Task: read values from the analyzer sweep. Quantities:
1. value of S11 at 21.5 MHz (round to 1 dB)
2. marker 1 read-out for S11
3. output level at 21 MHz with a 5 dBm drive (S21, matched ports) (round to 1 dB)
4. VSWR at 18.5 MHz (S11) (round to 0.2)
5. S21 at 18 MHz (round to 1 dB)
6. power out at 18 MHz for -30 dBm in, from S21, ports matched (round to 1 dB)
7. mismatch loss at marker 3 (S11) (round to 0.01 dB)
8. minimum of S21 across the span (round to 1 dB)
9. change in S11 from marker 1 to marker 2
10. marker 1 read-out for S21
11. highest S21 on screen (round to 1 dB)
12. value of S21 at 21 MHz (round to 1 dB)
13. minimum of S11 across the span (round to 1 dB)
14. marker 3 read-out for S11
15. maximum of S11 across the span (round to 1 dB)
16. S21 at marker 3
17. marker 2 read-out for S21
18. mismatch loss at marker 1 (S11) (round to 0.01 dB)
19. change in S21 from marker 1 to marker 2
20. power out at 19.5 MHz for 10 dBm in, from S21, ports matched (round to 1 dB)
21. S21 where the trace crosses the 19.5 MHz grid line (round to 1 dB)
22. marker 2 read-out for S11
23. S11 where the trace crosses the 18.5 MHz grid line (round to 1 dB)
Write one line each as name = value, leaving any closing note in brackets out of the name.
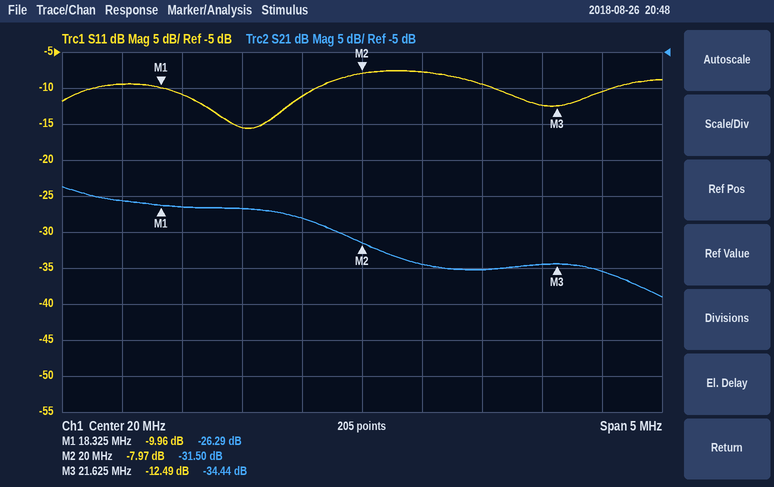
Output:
value of S11 at 21.5 MHz = -12 dB
marker 1 read-out for S11 = -9.96 dB
output level at 21 MHz with a 5 dBm drive (S21, matched ports) = -30 dBm
VSWR at 18.5 MHz (S11) = 1.8
S21 at 18 MHz = -26 dB
power out at 18 MHz for -30 dBm in, from S21, ports matched = -56 dBm
mismatch loss at marker 3 (S11) = 0.25 dB
minimum of S21 across the span = -39 dB
change in S11 from marker 1 to marker 2 = 1.99 dB
marker 1 read-out for S21 = -26.29 dB
highest S21 on screen = -24 dB
value of S21 at 21 MHz = -35 dB
minimum of S11 across the span = -16 dB
marker 3 read-out for S11 = -12.49 dB
maximum of S11 across the span = -8 dB
S21 at marker 3 = -34.44 dB
marker 2 read-out for S21 = -31.50 dB
mismatch loss at marker 1 (S11) = 0.46 dB
change in S21 from marker 1 to marker 2 = -5.21 dB
power out at 19.5 MHz for 10 dBm in, from S21, ports matched = -18 dBm
S21 where the trace crosses the 19.5 MHz grid line = -28 dB
marker 2 read-out for S11 = -7.97 dB
S11 where the trace crosses the 18.5 MHz grid line = -11 dB
